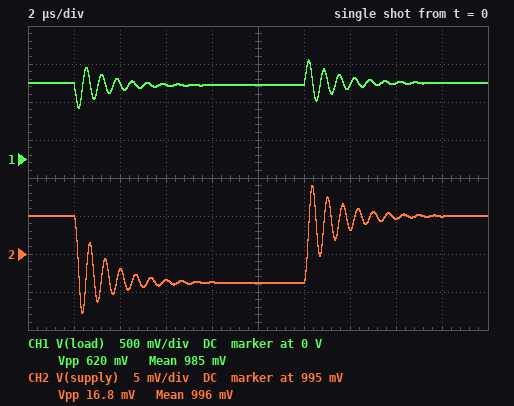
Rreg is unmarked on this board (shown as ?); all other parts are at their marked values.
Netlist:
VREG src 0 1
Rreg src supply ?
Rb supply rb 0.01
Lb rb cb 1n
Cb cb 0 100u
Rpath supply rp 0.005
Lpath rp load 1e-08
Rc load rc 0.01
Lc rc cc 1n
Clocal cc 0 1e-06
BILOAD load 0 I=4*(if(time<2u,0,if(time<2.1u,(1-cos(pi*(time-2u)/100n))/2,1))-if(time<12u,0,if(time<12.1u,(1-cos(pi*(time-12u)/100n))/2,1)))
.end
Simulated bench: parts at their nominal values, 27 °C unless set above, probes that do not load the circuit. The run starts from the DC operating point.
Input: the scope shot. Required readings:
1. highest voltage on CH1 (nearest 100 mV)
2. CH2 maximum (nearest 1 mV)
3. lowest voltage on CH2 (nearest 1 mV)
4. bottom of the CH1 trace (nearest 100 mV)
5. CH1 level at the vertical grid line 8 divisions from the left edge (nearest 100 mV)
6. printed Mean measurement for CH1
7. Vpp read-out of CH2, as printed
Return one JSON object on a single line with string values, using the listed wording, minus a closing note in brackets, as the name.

{"highest voltage on CH1": "1.3 V", "CH2 maximum": "1.004 V", "lowest voltage on CH2": "987 mV", "bottom of the CH1 trace": "700 mV", "CH1 level at the vertical grid line 8 divisions from the left edge": "1.0 V", "printed Mean measurement for CH1": "985 mV", "Vpp read-out of CH2, as printed": "16.8 mV"}
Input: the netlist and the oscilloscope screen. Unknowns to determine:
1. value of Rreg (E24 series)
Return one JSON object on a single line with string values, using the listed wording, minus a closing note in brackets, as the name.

{"value of Rreg": "2.2 mΩ"}
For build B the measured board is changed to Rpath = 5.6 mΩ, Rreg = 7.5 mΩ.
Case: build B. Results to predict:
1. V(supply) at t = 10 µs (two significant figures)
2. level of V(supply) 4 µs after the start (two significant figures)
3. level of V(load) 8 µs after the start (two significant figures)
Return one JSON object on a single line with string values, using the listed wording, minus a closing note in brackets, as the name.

{"V(supply) at t = 10 µs": "970 mV", "level of V(supply) 4 µs after the start": "980 mV", "level of V(load) 8 µs after the start": "950 mV"}
